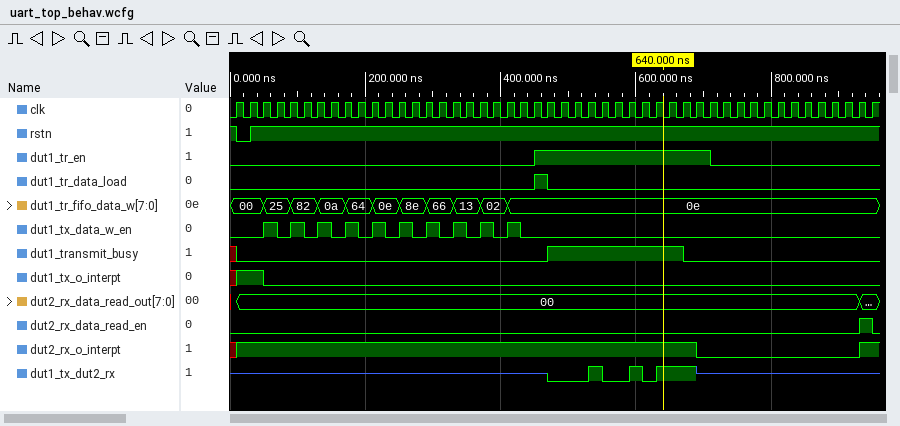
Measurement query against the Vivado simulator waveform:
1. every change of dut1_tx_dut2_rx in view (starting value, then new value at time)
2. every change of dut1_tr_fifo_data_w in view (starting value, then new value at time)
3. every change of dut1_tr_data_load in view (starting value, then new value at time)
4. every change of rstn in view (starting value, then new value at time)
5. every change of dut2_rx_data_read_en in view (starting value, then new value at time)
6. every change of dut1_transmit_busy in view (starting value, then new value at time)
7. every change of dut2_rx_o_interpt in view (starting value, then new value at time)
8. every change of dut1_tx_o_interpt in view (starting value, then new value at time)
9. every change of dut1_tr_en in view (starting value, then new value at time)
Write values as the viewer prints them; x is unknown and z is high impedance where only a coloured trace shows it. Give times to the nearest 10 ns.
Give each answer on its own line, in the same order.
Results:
z, 0 at 470 ns, 1 at 530 ns, 0 at 550 ns, 1 at 590 ns, 0 at 610 ns, 1 at 630 ns, z at 690 ns
00, 25 at 50 ns, 82 at 90 ns, 0a at 130 ns, 64 at 170 ns, 0e at 210 ns, 8e at 250 ns, 66 at 290 ns, 13 at 330 ns, 02 at 370 ns, 0e at 410 ns
0, 1 at 450 ns, 0 at 470 ns
1, 0 at 10 ns, 1 at 30 ns
0, 1 at 930 ns, 0 at 950 ns
x, 0 at 10 ns, 1 at 470 ns, 0 at 670 ns
x, 1 at 10 ns, 0 at 690 ns, 1 at 930 ns
x, 1 at 10 ns, 0 at 50 ns
0, 1 at 450 ns, 0 at 710 ns
